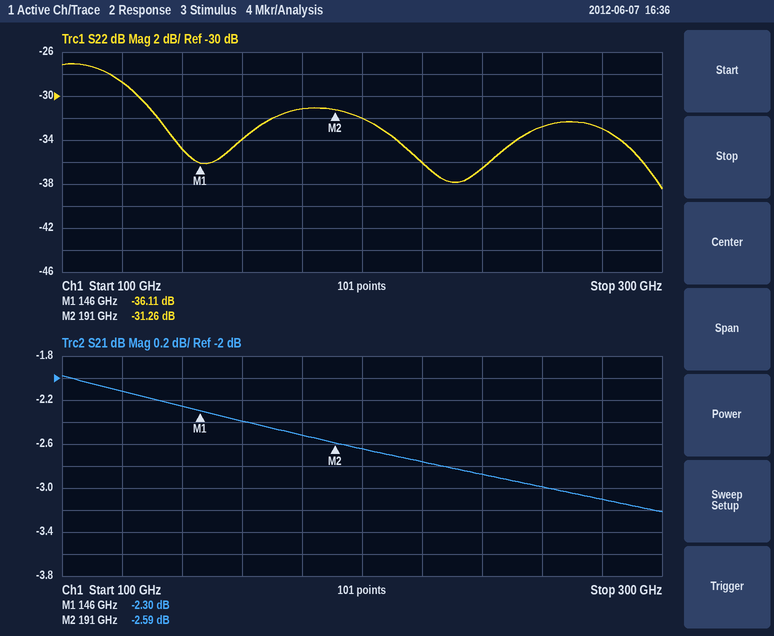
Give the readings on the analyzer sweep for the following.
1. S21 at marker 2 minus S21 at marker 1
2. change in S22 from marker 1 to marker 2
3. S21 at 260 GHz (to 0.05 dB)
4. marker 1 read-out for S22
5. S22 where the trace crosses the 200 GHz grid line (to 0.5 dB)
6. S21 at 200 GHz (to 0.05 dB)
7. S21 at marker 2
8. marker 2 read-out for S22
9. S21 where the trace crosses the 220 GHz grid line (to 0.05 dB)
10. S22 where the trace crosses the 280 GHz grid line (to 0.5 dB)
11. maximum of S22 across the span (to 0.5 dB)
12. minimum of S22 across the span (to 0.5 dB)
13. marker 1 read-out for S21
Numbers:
-0.29 dB
4.85 dB
-3.00 dB
-36.11 dB
-32.0 dB
-2.65 dB
-2.59 dB
-31.26 dB
-2.75 dB
-33.0 dB
-27.0 dB
-38.5 dB
-2.30 dB
